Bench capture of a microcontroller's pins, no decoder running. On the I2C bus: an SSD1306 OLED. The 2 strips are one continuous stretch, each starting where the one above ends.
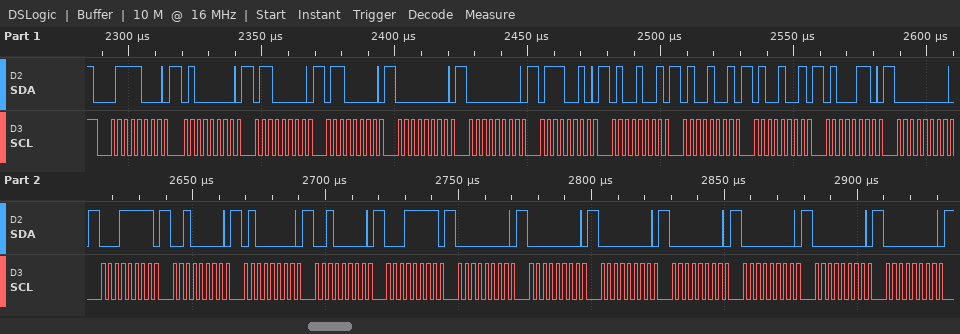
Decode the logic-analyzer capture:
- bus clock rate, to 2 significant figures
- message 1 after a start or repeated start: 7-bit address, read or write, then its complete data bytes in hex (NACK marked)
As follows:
400 kHz
0x3C write: 40 60 60 00 00 72 49 49 49 46 00 1F 20 40 20 1F 00 00 00 00 00 00 00
